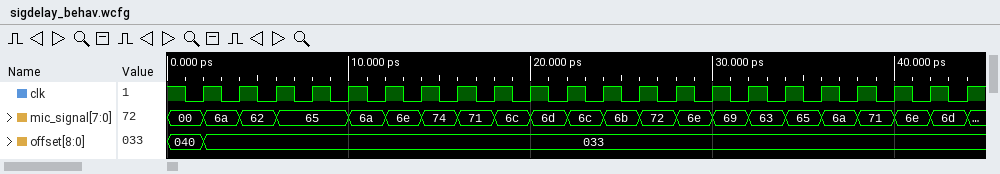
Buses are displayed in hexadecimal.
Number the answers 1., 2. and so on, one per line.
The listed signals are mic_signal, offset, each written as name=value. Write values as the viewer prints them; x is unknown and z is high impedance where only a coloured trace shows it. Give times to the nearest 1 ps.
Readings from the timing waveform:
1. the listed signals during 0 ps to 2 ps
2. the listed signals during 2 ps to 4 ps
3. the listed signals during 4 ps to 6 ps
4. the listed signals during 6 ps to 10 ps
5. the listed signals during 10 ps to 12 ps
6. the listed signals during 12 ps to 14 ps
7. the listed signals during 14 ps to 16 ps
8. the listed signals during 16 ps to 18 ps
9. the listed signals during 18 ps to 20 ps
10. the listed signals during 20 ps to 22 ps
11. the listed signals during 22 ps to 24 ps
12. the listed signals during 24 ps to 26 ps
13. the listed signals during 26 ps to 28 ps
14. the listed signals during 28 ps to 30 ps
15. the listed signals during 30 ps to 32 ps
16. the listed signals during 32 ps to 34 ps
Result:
1. mic_signal=00, offset=040
2. mic_signal=6a, offset=033
3. mic_signal=62, offset=033
4. mic_signal=65, offset=033
5. mic_signal=6a, offset=033
6. mic_signal=6e, offset=033
7. mic_signal=74, offset=033
8. mic_signal=71, offset=033
9. mic_signal=6c, offset=033
10. mic_signal=6d, offset=033
11. mic_signal=6c, offset=033
12. mic_signal=6b, offset=033
13. mic_signal=72, offset=033
14. mic_signal=6e, offset=033
15. mic_signal=69, offset=033
16. mic_signal=63, offset=033
